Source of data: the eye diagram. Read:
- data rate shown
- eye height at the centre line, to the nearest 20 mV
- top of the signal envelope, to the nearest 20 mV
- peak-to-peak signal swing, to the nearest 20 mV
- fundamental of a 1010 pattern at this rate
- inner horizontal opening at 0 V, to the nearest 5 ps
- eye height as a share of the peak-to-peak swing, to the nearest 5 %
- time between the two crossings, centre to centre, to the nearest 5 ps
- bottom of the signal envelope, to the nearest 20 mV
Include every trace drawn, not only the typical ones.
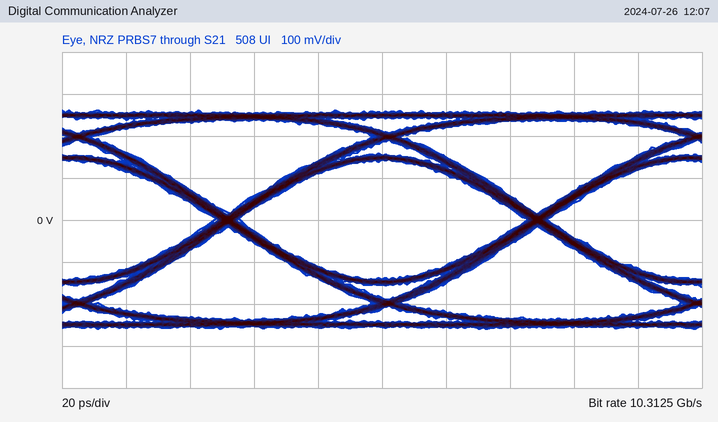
10.3125 Gb/s
280 mV
260 mV
520 mV
5.15625 GHz
90 ps
55 %
95 ps
-260 mV
